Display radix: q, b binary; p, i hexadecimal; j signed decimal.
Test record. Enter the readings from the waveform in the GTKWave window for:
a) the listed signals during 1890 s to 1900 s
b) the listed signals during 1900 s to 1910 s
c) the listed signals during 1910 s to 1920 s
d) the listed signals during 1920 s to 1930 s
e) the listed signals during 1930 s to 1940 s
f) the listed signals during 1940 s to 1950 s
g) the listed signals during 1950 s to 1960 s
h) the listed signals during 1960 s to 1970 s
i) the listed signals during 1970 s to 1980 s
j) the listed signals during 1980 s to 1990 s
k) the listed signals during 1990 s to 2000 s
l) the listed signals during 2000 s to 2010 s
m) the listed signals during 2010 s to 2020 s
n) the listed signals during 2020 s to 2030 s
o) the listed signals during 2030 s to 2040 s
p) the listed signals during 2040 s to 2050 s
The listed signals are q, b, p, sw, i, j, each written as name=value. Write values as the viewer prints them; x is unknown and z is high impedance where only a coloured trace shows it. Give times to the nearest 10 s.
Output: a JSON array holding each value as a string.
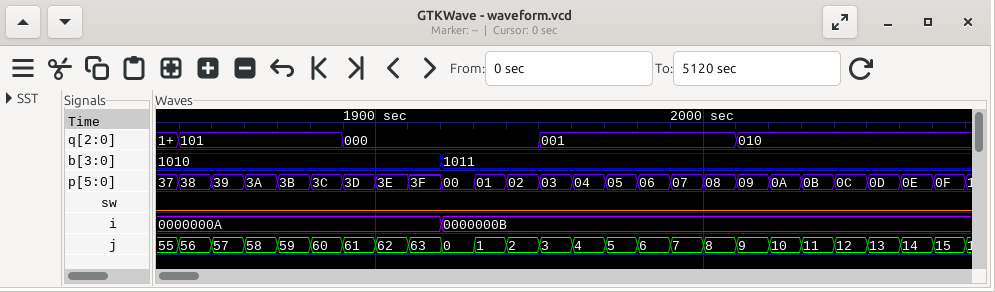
["q=000, b=1010, p=3D, sw=0, i=0000000A, j=61", "q=000, b=1010, p=3E, sw=0, i=0000000A, j=62", "q=000, b=1010, p=3F, sw=0, i=0000000A, j=63", "q=000, b=1011, p=00, sw=0, i=0000000B, j=0", "q=000, b=1011, p=01, sw=0, i=0000000B, j=1", "q=000, b=1011, p=02, sw=0, i=0000000B, j=2", "q=001, b=1011, p=03, sw=0, i=0000000B, j=3", "q=001, b=1011, p=04, sw=0, i=0000000B, j=4", "q=001, b=1011, p=05, sw=0, i=0000000B, j=5", "q=001, b=1011, p=06, sw=0, i=0000000B, j=6", "q=001, b=1011, p=07, sw=0, i=0000000B, j=7", "q=001, b=1011, p=08, sw=0, i=0000000B, j=8", "q=010, b=1011, p=09, sw=0, i=0000000B, j=9", "q=010, b=1011, p=0A, sw=0, i=0000000B, j=10", "q=010, b=1011, p=0B, sw=0, i=0000000B, j=11", "q=010, b=1011, p=0C, sw=0, i=0000000B, j=12"]
